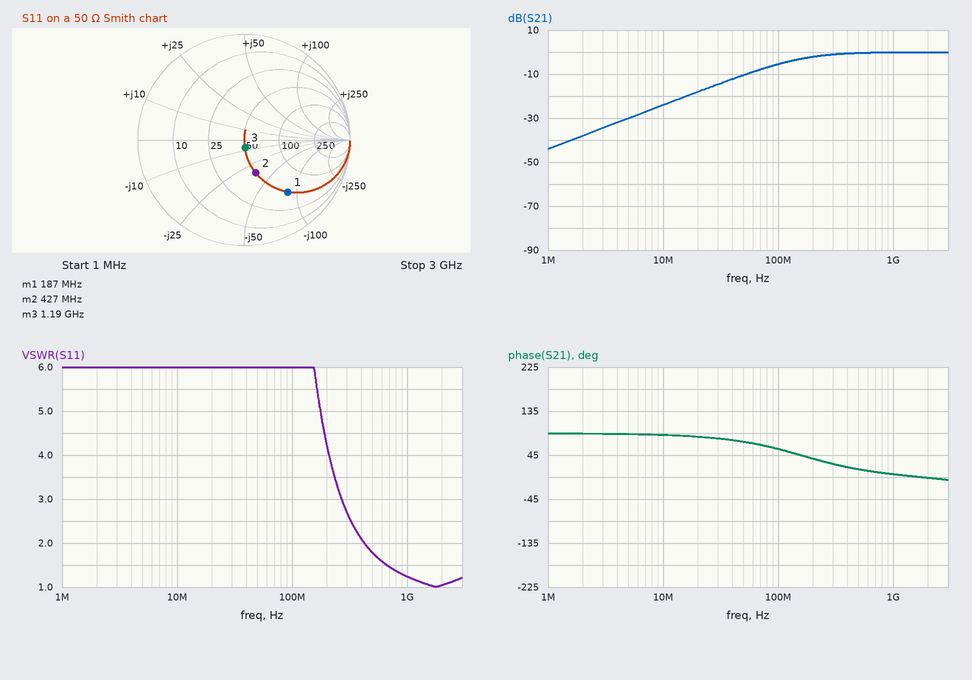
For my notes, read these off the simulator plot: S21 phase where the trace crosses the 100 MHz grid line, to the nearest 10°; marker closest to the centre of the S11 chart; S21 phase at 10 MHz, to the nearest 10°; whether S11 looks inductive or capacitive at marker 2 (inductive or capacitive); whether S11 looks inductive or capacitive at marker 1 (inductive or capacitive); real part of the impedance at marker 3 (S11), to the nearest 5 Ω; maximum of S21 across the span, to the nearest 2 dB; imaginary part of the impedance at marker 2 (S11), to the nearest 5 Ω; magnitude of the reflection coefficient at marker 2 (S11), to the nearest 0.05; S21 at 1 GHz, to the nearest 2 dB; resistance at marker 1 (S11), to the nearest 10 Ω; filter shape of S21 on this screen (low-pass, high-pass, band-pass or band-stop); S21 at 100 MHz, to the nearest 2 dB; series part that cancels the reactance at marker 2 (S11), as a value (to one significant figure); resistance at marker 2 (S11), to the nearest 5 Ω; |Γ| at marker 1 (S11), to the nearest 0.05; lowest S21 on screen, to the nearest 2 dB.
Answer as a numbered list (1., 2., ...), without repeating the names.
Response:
1. 60°
2. marker 3
3. 90°
4. capacitive
5. capacitive
6. 50 Ω
7. 0 dB
8. -35 Ω
9. 0.35
10. 0 dB
11. 50 Ω
12. high-pass
13. -6 dB
14. 10 nH
15. 50 Ω
16. 0.65
17. -44 dB
